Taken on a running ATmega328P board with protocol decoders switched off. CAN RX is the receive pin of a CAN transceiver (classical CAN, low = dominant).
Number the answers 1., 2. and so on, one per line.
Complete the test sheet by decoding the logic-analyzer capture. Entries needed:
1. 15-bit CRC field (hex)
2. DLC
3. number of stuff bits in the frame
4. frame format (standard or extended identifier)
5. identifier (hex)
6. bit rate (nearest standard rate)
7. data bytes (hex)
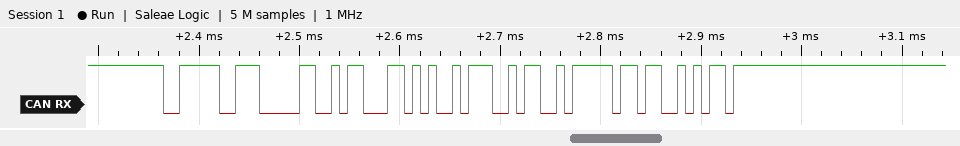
1. 0x7D95
2. 4
3. 3
4. standard
5. 0x3EE
6. 125 kbit/s
7. B1 A9 72 CB
